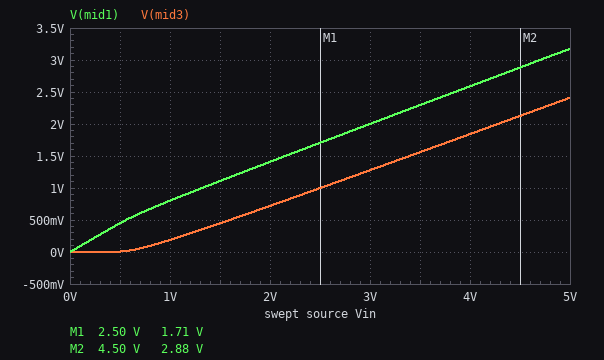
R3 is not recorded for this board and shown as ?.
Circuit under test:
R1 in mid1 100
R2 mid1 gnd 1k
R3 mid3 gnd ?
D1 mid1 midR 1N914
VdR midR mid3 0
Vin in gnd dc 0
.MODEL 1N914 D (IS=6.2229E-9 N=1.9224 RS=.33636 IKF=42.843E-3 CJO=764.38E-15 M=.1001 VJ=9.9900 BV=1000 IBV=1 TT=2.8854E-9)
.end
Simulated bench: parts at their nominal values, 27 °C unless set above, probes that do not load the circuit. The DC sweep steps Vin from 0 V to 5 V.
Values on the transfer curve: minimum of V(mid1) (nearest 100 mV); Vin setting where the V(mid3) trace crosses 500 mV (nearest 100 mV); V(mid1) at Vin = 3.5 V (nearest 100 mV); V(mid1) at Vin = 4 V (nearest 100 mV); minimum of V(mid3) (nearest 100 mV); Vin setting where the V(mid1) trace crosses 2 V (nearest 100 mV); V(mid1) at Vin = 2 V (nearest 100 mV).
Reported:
0 V
1.6 V
2.3 V
2.6 V
0 V
3.0 V
1.4 V
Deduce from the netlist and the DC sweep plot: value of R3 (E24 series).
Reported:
160 Ω
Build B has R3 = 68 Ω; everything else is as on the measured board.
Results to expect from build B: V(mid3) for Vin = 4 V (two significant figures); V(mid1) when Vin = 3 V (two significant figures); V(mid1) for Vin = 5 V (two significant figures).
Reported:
1.2 V
1.6 V
2.4 V
